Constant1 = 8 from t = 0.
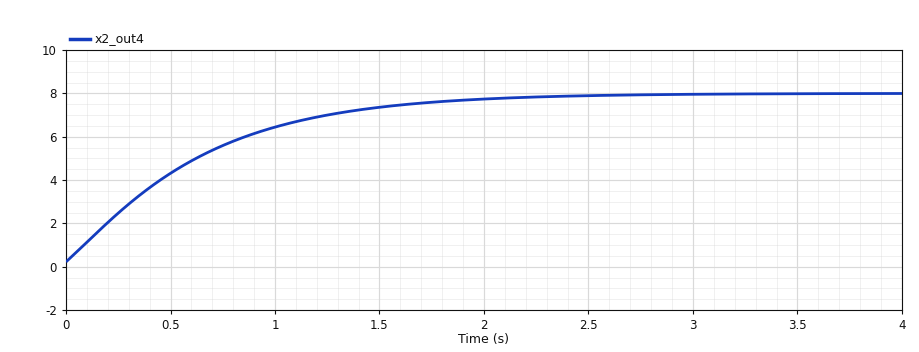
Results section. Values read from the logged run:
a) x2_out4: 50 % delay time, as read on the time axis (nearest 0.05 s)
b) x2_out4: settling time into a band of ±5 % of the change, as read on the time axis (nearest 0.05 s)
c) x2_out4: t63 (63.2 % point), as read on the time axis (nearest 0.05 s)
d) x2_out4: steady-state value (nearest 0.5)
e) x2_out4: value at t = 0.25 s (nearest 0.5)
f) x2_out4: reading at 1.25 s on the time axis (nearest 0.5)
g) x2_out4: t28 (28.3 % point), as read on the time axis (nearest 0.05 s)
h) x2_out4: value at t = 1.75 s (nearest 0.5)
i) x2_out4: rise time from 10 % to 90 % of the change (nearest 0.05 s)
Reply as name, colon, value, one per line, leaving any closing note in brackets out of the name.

x2_out4: 50 % delay time, as read on the time axis: 0.45 s
x2_out4: settling time into a band of ±5 % of the change, as read on the time axis: 1.80 s
x2_out4: t63 (63.2 % point), as read on the time axis: 0.65 s
x2_out4: steady-state value: 8.0
x2_out4: value at t = 0.25 s: 2.5
x2_out4: reading at 1.25 s on the time axis: 7.0
x2_out4: t28 (28.3 % point), as read on the time axis: 0.25 s
x2_out4: value at t = 1.75 s: 7.5
x2_out4: rise time from 10 % to 90 % of the change: 1.30 s
